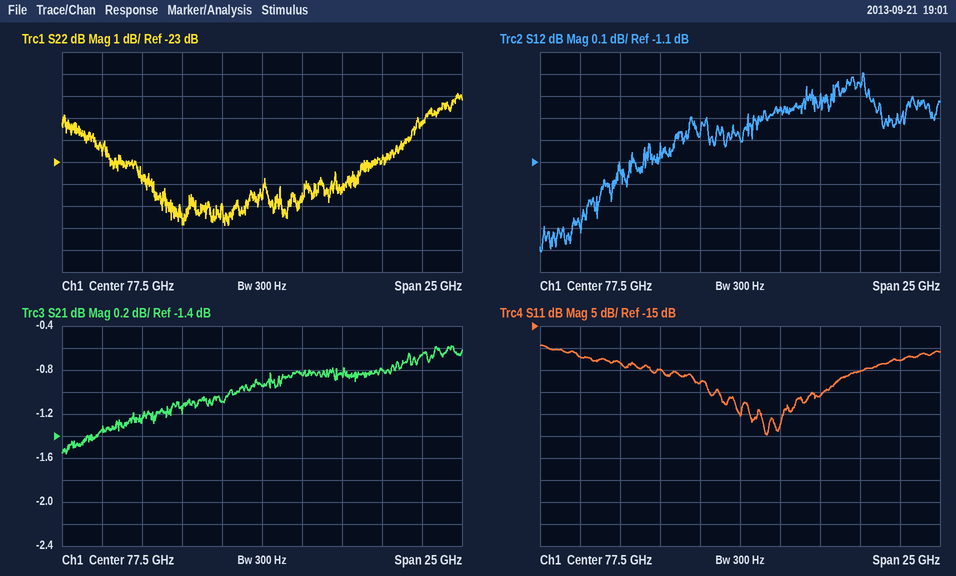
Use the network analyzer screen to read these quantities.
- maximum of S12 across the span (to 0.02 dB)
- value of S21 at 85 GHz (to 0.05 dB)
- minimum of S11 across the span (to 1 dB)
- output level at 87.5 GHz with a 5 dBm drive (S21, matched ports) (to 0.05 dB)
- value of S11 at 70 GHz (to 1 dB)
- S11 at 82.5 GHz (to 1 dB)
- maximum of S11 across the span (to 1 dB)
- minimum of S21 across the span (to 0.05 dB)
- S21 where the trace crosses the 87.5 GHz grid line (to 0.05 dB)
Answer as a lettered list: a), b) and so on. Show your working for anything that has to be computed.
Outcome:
a) -0.70 dB
b) -0.80 dB
c) -40 dB
d) 5 dBm + (-0.65 dB) = 4.35 dBm
e) -23 dB
f) -31 dB
g) -19 dB
h) -1.55 dB
i) -0.65 dB
